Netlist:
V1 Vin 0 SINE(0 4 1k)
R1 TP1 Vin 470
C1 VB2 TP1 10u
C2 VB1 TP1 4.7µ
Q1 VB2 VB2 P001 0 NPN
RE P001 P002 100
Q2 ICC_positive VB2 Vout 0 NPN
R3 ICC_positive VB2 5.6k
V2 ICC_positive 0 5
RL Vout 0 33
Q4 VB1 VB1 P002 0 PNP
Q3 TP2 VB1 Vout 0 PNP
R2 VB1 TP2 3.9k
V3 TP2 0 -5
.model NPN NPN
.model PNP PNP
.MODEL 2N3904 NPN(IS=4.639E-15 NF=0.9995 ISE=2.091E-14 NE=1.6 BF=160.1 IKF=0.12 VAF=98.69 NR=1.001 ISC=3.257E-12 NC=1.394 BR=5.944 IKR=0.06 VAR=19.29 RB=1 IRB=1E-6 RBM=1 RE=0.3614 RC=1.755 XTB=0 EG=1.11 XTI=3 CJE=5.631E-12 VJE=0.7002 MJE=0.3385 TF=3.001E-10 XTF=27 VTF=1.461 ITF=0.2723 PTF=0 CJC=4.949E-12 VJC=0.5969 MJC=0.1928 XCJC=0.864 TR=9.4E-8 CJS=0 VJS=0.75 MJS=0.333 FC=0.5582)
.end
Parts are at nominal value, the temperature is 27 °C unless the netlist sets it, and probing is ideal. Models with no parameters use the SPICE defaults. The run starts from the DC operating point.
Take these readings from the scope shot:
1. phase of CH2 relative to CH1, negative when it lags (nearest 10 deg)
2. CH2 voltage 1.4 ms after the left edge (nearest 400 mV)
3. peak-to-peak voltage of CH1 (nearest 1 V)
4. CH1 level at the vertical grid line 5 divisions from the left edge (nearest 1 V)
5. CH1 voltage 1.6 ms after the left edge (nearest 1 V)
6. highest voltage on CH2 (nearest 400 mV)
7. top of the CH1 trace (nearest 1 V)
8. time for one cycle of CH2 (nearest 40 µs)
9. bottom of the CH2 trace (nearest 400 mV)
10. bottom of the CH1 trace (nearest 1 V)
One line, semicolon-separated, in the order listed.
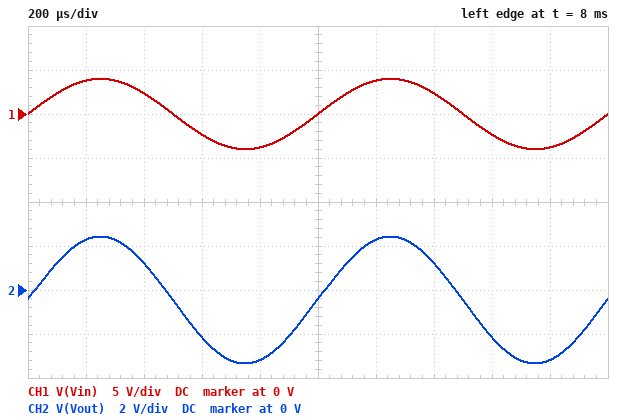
0 deg; 1.2 V; 8 V; 0 V; -2 V; 2.4 V; 4 V; 1.00 ms; -3.2 V; -4 V
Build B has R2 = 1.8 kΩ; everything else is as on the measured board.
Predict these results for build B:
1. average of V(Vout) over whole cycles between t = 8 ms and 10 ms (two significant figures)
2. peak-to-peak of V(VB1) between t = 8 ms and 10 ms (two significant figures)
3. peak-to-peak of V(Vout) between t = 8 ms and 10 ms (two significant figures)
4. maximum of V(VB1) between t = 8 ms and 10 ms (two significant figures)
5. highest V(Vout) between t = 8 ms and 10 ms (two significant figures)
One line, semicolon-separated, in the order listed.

-1.5 V; 5.4 V; 5.3 V; 320 mV; 1.1 V
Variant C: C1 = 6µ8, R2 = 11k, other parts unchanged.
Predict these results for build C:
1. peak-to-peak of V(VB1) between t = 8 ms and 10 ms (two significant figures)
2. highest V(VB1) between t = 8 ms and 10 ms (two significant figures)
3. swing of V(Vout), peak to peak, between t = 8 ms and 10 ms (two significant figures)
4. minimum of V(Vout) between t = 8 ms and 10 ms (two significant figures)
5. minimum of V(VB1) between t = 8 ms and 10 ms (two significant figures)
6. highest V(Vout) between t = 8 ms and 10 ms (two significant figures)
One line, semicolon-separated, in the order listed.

6.3 V; 3.1 V; 6.1 V; -2.4 V; -3.3 V; 3.7 V
